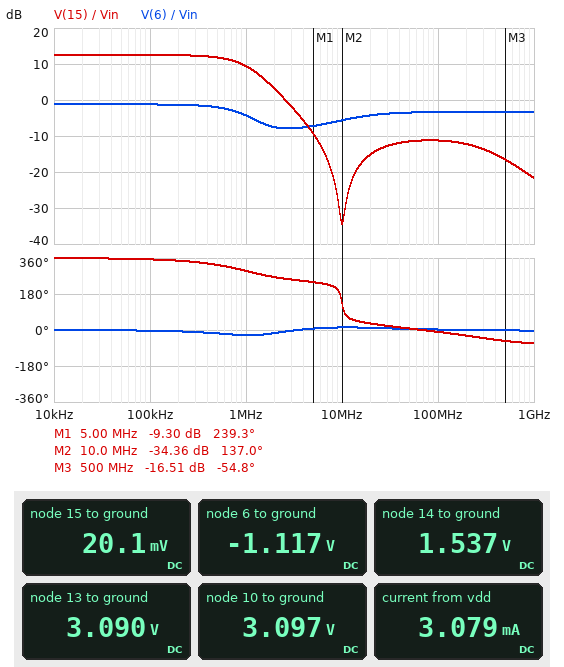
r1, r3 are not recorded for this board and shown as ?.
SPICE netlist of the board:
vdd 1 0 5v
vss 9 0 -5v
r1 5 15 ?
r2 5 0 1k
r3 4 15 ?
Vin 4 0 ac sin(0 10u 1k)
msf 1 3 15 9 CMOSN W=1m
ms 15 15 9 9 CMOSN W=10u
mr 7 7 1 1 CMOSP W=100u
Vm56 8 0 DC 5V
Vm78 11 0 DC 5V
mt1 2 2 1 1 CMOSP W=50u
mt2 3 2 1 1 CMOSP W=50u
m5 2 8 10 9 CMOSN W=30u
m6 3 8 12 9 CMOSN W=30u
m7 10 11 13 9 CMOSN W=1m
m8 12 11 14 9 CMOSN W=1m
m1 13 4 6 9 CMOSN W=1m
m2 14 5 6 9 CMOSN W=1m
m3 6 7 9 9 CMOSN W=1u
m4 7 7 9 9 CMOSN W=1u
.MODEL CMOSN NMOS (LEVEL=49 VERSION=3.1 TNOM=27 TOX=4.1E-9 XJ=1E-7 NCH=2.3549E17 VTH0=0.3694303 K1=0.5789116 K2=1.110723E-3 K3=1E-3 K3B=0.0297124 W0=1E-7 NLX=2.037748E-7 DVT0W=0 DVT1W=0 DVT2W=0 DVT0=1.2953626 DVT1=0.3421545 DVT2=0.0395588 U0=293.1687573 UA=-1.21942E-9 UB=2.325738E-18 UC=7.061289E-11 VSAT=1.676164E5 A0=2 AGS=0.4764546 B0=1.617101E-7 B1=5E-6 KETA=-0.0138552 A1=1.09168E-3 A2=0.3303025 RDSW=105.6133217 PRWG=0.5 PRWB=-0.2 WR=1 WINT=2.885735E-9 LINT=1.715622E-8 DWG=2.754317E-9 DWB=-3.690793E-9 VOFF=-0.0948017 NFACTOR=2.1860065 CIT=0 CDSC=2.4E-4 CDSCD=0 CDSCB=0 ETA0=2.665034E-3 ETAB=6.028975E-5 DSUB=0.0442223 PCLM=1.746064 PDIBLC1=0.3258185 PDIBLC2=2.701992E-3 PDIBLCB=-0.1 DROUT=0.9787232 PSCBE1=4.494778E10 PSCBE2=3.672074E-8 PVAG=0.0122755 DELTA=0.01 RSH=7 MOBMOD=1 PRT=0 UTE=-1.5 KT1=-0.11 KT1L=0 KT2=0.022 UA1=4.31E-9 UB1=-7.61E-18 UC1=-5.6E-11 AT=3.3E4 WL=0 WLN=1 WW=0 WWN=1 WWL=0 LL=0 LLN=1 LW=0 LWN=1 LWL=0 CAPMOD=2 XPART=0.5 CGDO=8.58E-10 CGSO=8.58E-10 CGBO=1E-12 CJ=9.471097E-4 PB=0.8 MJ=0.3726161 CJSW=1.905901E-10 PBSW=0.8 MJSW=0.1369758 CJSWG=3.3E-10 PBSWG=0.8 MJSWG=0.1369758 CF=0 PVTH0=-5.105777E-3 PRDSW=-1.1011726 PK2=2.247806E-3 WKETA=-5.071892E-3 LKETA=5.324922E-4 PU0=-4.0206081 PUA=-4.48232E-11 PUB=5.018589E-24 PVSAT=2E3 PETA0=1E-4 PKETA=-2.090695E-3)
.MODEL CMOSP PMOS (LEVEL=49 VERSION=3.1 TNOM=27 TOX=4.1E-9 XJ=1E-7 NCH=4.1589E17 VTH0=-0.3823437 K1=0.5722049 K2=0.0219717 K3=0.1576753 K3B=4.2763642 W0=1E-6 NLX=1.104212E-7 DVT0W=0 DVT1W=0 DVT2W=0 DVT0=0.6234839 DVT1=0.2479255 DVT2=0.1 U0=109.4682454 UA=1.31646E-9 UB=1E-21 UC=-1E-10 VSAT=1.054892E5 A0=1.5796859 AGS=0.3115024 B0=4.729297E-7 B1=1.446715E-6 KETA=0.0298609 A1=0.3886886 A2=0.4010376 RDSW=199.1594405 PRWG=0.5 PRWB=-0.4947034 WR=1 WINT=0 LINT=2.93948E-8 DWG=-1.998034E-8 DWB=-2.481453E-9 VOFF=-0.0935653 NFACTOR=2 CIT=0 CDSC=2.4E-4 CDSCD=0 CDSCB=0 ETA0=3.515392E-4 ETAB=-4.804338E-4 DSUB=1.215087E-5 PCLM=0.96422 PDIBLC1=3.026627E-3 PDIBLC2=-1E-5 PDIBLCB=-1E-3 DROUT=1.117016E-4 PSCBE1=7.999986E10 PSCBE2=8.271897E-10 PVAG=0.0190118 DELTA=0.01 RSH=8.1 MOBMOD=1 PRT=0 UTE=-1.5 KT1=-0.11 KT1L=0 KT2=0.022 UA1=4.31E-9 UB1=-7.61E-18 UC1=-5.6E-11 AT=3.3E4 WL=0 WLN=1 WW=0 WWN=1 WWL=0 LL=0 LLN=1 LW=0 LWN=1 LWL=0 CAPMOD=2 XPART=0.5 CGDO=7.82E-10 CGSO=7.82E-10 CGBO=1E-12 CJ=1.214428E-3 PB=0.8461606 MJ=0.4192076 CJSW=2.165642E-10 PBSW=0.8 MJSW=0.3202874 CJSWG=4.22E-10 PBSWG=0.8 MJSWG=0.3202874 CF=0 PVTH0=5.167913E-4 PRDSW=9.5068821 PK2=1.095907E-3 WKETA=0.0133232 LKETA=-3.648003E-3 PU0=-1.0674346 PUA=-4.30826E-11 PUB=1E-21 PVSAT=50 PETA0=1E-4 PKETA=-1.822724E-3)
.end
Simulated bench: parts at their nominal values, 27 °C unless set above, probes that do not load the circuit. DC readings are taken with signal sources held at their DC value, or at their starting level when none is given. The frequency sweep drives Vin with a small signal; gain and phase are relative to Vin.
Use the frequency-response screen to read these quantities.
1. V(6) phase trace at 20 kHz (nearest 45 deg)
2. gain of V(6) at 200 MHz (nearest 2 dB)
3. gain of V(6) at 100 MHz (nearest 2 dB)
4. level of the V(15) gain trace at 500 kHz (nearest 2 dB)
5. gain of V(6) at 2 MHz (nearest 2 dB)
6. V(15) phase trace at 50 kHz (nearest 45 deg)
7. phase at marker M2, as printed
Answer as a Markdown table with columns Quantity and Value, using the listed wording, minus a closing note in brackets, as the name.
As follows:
| Quantity | Value |
|---|---|
| V(6) phase trace at 20 kHz | 0 deg |
| gain of V(6) at 200 MHz | -4 dB |
| gain of V(6) at 100 MHz | -4 dB |
| level of the V(15) gain trace at 500 kHz | 12 dB |
| gain of V(6) at 2 MHz | -8 dB |
| V(15) phase trace at 50 kHz | 360 deg |
| phase at marker M2, as printed | 137.0 deg |
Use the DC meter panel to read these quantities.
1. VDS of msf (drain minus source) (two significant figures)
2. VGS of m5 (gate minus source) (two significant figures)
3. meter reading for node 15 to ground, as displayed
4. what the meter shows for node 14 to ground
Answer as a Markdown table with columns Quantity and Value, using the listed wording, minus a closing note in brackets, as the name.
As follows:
| Quantity | Value |
|---|---|
| VDS of msf (drain minus source) | 5.0 V |
| VGS of m5 (gate minus source) | 1.9 V |
| meter reading for node 15 to ground, as displayed | 20.1 mV |
| what the meter shows for node 14 to ground | 1.537 V |
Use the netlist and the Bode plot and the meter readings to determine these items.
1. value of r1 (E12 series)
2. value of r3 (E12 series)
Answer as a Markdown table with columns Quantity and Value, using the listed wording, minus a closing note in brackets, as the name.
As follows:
| Quantity | Value |
|---|---|
| value of r1 | 3.3 kΩ |
| value of r3 | 680 Ω |
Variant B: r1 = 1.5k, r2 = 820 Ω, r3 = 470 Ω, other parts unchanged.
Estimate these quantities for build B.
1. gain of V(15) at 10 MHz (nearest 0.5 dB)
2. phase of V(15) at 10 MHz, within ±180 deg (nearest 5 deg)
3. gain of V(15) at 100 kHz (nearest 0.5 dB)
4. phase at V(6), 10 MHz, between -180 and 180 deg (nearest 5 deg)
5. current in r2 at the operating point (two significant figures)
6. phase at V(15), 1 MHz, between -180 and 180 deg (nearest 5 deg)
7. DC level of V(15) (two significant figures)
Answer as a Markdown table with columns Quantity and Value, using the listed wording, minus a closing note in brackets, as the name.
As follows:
| Quantity | Value |
|---|---|
| gain of V(15) at 10 MHz | -26.5 dB |
| phase of V(15) at 10 MHz, within ±180 deg | 30 deg |
| gain of V(15) at 100 kHz | 9.0 dB |
| phase at V(6), 10 MHz, between -180 and 180 deg | 10 deg |
| current in r2 at the operating point | 5.7 µA |
| phase at V(15), 1 MHz, between -180 and 180 deg | -50 deg |
| DC level of V(15) | 13 mV |
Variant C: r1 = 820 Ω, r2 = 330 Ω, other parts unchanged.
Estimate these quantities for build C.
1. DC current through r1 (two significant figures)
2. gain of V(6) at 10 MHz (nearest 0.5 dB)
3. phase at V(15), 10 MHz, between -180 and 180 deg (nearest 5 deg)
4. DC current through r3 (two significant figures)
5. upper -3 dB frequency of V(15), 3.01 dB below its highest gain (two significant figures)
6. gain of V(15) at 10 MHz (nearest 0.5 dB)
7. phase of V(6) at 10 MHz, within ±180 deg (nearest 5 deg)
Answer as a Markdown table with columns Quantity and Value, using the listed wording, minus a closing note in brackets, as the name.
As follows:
| Quantity | Value |
|---|---|
| DC current through r1 | 14 µA |
| gain of V(6) at 10 MHz | -7.0 dB |
| phase at V(15), 10 MHz, between -180 and 180 deg | -140 deg |
| DC current through r3 | 24 µA |
| upper -3 dB frequency of V(15), 3.01 dB below its highest gain | 1.1 MHz |
| gain of V(15) at 10 MHz | -28.5 dB |
| phase of V(6) at 10 MHz, within ±180 deg | 5 deg |
